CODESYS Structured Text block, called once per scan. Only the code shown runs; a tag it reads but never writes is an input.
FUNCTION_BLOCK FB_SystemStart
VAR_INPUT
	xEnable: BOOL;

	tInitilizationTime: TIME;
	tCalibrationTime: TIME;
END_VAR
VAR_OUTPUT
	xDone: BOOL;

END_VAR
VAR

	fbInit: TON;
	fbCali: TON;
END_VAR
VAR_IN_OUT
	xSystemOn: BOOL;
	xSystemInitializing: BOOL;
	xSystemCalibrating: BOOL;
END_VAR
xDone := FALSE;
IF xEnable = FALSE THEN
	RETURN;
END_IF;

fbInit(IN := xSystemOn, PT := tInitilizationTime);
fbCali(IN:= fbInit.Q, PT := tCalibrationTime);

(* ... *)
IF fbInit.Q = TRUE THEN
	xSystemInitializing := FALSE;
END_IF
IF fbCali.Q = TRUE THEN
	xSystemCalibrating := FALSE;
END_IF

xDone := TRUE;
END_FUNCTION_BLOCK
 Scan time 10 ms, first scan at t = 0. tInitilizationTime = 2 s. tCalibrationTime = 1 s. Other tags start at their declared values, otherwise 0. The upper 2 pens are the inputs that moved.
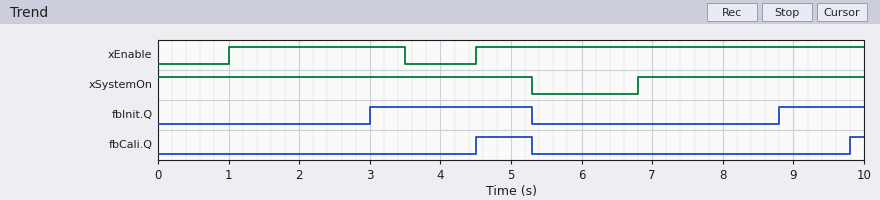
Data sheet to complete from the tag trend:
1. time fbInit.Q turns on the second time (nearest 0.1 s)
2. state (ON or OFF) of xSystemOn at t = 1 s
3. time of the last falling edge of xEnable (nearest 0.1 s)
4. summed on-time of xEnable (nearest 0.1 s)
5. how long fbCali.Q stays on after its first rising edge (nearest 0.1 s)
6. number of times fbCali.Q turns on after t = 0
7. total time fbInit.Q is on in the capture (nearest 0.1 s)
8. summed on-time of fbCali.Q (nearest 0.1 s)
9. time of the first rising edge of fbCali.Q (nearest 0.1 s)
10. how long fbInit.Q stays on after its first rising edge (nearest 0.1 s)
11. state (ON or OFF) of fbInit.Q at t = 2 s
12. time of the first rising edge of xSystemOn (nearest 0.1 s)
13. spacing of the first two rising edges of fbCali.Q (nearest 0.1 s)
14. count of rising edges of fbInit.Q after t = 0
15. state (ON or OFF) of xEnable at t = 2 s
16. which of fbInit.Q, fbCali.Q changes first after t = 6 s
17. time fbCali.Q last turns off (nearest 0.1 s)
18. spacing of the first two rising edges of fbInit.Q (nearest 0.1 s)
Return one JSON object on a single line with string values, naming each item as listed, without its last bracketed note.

{"time fbInit.Q turns on the second time": "8.8 s", "state (ON or OFF) of xSystemOn at t = 1 s": "ON", "time of the last falling edge of xEnable": "3.5 s", "summed on-time of xEnable": "8.0 s", "how long fbCali.Q stays on after its first rising edge": "0.8 s", "number of times fbCali.Q turns on after t = 0": "2", "total time fbInit.Q is on in the capture": "3.5 s", "summed on-time of fbCali.Q": "1.0 s", "time of the first rising edge of fbCali.Q": "4.5 s", "how long fbInit.Q stays on after its first rising edge": "2.3 s", "state (ON or OFF) of fbInit.Q at t = 2 s": "OFF", "time of the first rising edge of xSystemOn": "6.8 s", "spacing of the first two rising edges of fbCali.Q": "5.3 s", "count of rising edges of fbInit.Q after t = 0": "2", "state (ON or OFF) of xEnable at t = 2 s": "ON", "which of fbInit.Q, fbCali.Q changes first after t = 6 s": "fbInit.Q", "time fbCali.Q last turns off": "5.3 s", "spacing of the first two rising edges of fbInit.Q": "5.8 s"}
